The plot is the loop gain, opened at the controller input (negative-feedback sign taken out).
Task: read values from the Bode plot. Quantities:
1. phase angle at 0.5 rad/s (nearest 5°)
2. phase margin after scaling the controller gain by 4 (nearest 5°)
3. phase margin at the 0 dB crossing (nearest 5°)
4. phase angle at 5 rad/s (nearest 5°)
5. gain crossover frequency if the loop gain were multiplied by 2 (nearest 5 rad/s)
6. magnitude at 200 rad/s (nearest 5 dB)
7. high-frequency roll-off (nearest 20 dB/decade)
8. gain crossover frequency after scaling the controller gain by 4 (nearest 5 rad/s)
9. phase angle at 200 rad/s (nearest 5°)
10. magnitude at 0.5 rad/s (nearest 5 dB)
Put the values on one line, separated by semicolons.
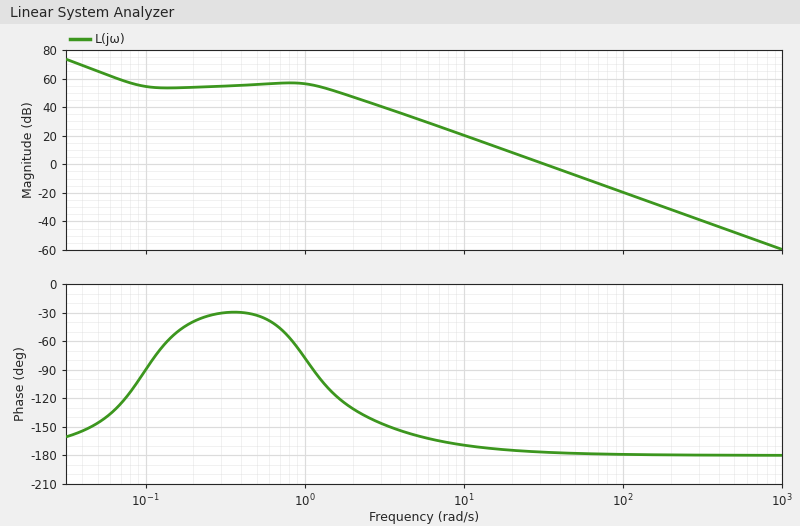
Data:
-35°; 0°; 5°; -160°; 45 rad/s; -30 dB; -40 dB/decade; 65 rad/s; -180°; 55 dB
